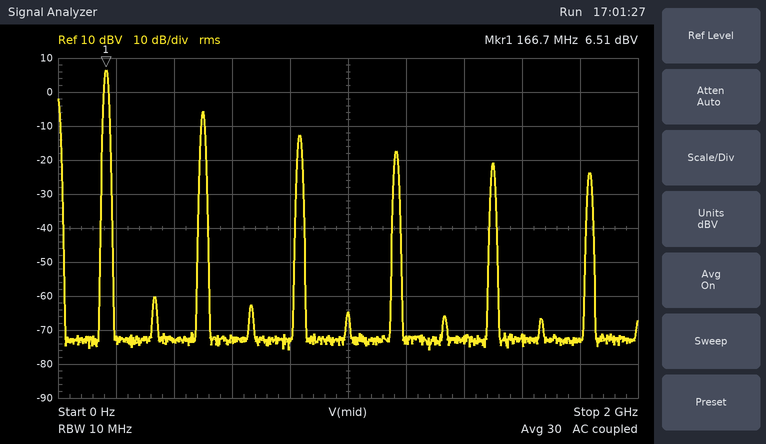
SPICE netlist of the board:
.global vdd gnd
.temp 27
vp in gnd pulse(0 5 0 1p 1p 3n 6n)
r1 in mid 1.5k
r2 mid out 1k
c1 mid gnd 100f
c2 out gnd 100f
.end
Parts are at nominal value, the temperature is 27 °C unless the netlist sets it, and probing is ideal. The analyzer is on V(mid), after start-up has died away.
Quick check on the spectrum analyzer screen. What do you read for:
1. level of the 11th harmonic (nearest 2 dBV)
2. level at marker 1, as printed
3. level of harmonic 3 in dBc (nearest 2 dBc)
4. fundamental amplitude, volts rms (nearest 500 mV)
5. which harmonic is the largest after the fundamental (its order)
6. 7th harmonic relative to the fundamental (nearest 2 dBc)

-24 dBV
6.51 dBV
-12 dBc
2.0 V
3
-24 dBc
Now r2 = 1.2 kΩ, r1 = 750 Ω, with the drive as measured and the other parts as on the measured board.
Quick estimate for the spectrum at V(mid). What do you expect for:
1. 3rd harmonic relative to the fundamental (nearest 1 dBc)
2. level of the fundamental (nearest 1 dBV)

-11 dBc
7 dBV
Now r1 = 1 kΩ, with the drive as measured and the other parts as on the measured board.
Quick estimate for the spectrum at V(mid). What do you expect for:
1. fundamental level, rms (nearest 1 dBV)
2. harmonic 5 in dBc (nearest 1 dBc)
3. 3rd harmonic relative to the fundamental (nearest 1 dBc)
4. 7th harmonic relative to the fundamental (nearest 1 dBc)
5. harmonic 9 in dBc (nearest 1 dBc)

7 dBV
-17 dBc
-11 dBc
-22 dBc
-25 dBc
